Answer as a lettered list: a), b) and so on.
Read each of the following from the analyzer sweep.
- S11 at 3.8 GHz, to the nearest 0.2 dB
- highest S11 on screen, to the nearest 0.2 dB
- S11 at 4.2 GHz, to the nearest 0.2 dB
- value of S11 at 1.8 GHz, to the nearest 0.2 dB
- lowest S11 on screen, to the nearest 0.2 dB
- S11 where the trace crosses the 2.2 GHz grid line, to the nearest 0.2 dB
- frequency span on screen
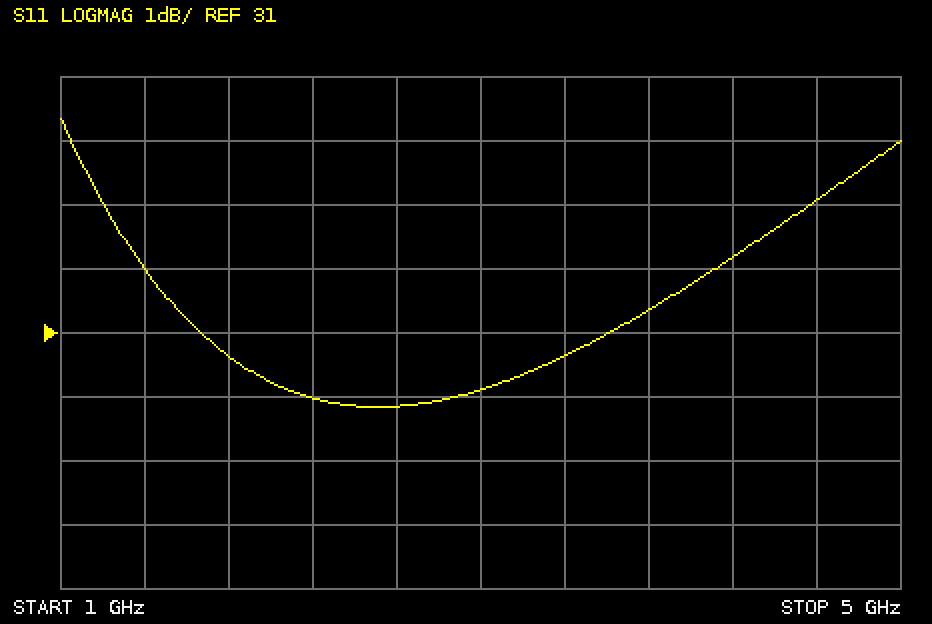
a) 31.4 dB
b) 34.4 dB
c) 32.2 dB
d) 30.6 dB
e) 29.8 dB
f) 30.0 dB
g) 4 GHz
